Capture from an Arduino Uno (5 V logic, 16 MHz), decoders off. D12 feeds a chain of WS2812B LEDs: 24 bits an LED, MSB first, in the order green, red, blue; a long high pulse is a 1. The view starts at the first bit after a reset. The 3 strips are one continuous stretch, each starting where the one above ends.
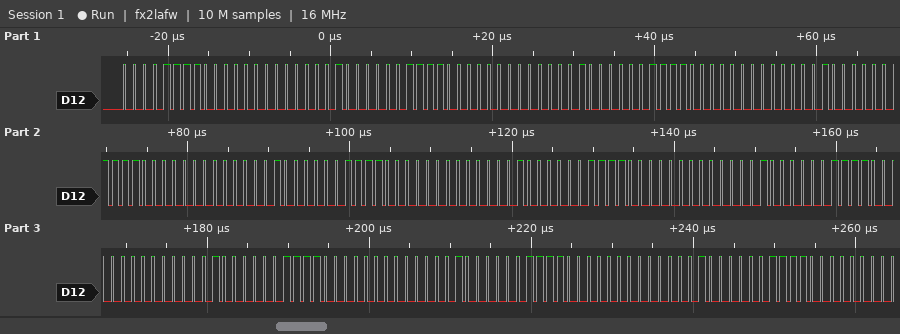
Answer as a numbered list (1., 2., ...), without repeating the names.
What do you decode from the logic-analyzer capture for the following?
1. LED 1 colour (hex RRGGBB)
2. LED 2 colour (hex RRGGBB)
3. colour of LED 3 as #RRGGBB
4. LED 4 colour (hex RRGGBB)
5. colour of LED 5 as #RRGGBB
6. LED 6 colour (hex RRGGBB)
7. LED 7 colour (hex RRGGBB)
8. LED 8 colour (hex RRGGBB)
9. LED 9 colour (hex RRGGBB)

1. #000F04
2. #000F04
3. #000F04
4. #000F04
5. #000F04
6. #000F04
7. #000F04
8. #000F04
9. #000F04
